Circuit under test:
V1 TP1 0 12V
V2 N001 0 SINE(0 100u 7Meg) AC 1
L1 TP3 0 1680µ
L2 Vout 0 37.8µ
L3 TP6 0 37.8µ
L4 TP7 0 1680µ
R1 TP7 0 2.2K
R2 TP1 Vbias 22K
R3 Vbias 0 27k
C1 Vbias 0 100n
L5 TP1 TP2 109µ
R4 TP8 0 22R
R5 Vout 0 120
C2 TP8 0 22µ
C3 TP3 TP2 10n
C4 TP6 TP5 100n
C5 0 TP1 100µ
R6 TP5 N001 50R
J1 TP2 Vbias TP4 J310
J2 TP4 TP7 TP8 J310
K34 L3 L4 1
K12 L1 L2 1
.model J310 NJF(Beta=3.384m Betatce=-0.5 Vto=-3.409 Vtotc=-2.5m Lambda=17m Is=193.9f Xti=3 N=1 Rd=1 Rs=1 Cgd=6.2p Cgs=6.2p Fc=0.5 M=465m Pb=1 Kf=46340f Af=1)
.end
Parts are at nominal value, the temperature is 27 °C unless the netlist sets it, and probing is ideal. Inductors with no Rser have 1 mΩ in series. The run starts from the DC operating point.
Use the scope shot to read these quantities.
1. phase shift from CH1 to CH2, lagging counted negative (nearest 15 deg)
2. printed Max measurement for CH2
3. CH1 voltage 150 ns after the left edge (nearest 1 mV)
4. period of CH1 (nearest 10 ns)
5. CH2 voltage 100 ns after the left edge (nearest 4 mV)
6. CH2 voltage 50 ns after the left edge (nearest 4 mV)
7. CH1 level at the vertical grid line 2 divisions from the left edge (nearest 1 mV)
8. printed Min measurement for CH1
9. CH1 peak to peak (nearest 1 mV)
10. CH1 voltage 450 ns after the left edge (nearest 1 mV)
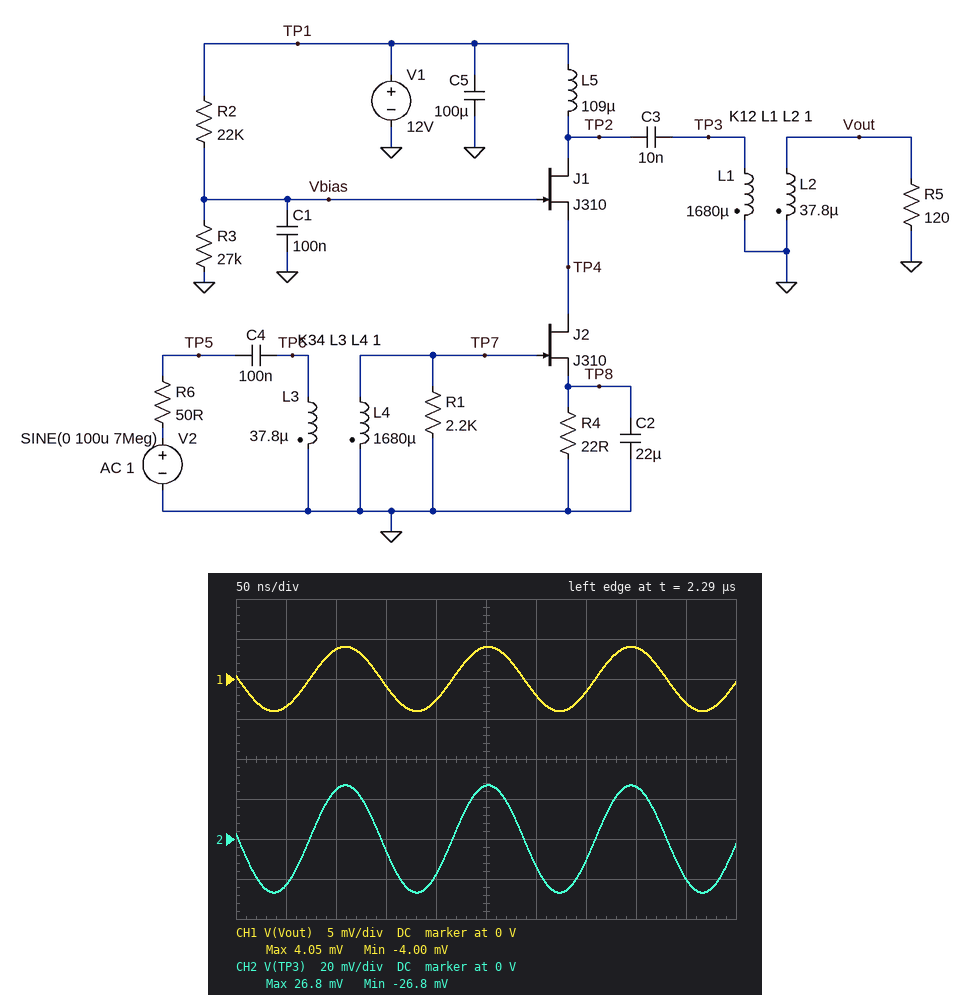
0 deg
26.8 mV
-1 mV
140 ns
24 mV
-24 mV
4 mV
-4.00 mV
8 mV
-3 mV
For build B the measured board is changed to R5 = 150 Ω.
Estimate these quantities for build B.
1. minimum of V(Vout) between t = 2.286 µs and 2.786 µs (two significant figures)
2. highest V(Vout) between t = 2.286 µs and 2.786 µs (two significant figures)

-4.8 mV
4.8 mV
